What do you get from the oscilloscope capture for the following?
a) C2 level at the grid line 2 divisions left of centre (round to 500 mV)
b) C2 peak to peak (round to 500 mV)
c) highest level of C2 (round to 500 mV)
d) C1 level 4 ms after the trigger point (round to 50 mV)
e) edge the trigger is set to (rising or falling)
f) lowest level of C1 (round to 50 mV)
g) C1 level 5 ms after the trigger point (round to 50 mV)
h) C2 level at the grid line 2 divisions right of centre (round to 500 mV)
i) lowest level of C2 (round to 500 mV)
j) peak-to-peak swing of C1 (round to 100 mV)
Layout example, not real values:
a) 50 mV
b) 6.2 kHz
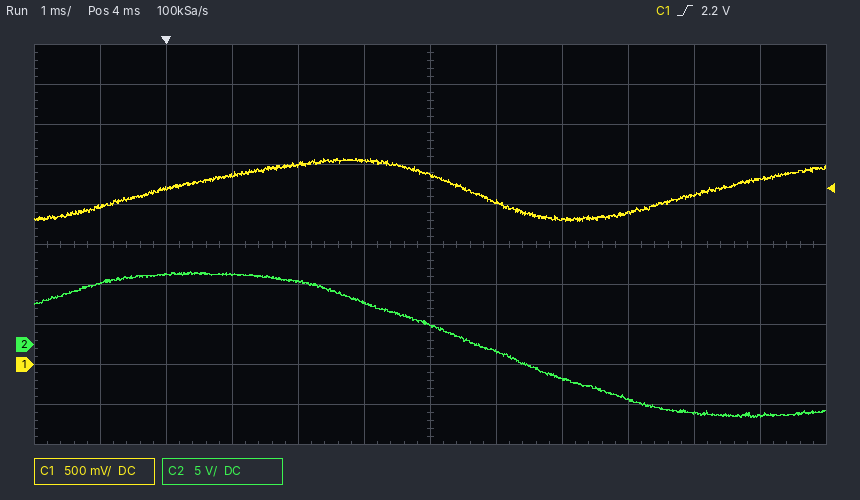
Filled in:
a) 8.0 V
b) 18.0 V
c) 9.0 V
d) 2.35 V
e) rising
f) 1.80 V
g) 2.05 V
h) -4.5 V
i) -9.0 V
j) 800 mV
